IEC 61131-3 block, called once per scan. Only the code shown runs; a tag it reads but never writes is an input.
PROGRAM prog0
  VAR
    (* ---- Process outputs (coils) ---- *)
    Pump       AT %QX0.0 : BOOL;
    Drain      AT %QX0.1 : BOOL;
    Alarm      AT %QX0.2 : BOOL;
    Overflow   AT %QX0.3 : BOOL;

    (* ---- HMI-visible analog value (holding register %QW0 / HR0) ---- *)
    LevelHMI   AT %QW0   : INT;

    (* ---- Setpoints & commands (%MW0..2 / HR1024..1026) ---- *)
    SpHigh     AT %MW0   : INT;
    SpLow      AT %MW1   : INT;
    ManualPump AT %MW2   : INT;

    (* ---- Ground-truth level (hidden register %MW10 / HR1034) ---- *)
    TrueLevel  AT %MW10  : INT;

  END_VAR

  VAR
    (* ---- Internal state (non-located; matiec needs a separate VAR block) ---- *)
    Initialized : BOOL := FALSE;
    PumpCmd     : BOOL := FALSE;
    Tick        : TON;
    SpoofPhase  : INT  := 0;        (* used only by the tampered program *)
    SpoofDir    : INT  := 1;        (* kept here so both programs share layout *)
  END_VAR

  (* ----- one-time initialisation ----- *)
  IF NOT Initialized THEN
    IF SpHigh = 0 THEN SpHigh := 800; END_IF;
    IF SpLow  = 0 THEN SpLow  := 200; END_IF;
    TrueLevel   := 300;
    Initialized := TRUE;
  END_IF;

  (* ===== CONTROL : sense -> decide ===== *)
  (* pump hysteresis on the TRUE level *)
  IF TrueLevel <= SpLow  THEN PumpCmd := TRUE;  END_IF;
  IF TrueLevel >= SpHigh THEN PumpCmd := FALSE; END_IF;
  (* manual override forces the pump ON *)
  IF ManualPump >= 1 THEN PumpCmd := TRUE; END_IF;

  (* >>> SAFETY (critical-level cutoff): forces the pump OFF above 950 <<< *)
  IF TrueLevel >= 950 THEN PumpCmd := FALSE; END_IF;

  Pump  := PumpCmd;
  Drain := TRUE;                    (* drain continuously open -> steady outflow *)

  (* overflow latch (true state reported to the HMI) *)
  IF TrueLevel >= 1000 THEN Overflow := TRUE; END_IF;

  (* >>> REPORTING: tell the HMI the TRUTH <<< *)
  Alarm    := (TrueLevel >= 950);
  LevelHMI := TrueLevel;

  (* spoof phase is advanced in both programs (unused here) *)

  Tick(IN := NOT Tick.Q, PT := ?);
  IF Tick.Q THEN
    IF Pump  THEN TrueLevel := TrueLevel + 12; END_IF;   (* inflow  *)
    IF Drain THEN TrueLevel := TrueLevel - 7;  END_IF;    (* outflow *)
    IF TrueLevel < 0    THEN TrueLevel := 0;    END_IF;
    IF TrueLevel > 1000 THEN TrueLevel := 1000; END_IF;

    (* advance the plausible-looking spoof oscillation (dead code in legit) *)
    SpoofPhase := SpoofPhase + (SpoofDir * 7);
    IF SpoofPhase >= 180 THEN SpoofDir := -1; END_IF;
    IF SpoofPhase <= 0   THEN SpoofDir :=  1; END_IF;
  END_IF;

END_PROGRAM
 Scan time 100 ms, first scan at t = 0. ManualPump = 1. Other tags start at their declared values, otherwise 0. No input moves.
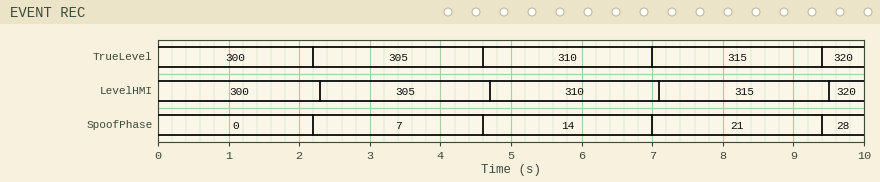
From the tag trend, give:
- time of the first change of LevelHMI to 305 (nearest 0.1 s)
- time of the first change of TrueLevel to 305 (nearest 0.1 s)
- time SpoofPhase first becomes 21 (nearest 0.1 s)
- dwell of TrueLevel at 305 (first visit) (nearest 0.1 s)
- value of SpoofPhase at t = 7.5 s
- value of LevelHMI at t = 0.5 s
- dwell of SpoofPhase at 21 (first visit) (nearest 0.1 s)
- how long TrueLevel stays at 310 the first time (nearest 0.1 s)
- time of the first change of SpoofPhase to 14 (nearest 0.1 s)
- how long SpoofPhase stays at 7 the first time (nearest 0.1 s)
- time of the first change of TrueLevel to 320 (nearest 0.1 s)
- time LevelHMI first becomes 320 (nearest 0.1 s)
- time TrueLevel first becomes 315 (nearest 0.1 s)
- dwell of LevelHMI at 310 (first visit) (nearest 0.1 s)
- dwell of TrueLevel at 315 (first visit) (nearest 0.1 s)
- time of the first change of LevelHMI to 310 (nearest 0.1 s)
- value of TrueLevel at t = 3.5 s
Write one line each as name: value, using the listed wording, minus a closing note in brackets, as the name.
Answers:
time of the first change of LevelHMI to 305: 2.3 s
time of the first change of TrueLevel to 305: 2.2 s
time SpoofPhase first becomes 21: 7.0 s
dwell of TrueLevel at 305 (first visit): 2.4 s
value of SpoofPhase at t = 7.5 s: 21
value of LevelHMI at t = 0.5 s: 300
dwell of SpoofPhase at 21 (first visit): 2.4 s
how long TrueLevel stays at 310 the first time: 2.4 s
time of the first change of SpoofPhase to 14: 4.6 s
how long SpoofPhase stays at 7 the first time: 2.4 s
time of the first change of TrueLevel to 320: 9.4 s
time LevelHMI first becomes 320: 9.5 s
time TrueLevel first becomes 315: 7.0 s
dwell of LevelHMI at 310 (first visit): 2.4 s
dwell of TrueLevel at 315 (first visit): 2.4 s
time of the first change of LevelHMI to 310: 4.7 s
value of TrueLevel at t = 3.5 s: 305
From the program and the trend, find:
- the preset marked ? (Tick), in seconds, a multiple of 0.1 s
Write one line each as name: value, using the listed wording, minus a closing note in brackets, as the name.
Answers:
the preset marked ? (Tick), in seconds, a multiple of 0.1 s: 2.2 s
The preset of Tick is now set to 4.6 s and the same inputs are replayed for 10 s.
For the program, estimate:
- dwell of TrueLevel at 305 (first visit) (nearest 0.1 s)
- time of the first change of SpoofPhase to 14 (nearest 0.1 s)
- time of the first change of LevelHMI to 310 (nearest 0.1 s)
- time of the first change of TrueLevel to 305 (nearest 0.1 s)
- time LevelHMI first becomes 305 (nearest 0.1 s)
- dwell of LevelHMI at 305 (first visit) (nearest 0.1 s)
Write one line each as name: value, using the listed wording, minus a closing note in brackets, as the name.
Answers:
dwell of TrueLevel at 305 (first visit): 4.8 s
time of the first change of SpoofPhase to 14: 9.4 s
time of the first change of LevelHMI to 310: 9.5 s
time of the first change of TrueLevel to 305: 4.6 s
time LevelHMI first becomes 305: 4.7 s
dwell of LevelHMI at 305 (first visit): 4.8 s
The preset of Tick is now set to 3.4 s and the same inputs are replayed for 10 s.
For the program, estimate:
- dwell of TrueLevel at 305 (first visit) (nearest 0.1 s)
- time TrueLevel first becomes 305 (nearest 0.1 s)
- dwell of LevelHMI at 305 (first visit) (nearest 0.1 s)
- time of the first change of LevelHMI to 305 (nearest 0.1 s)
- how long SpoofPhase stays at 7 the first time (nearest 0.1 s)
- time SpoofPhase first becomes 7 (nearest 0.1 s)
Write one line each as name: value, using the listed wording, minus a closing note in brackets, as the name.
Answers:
dwell of TrueLevel at 305 (first visit): 3.6 s
time TrueLevel first becomes 305: 3.4 s
dwell of LevelHMI at 305 (first visit): 3.6 s
time of the first change of LevelHMI to 305: 3.5 s
how long SpoofPhase stays at 7 the first time: 3.6 s
time SpoofPhase first becomes 7: 3.4 s
